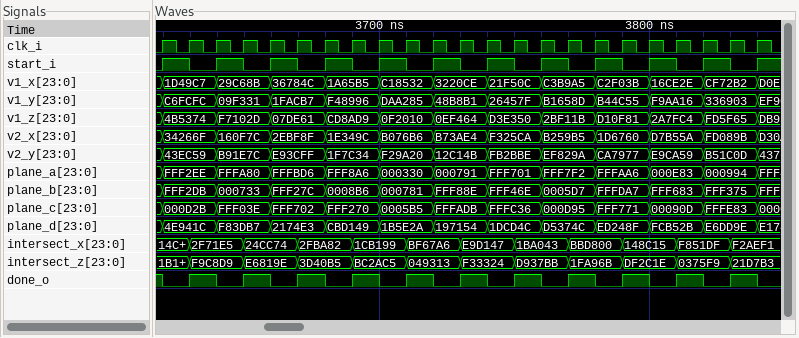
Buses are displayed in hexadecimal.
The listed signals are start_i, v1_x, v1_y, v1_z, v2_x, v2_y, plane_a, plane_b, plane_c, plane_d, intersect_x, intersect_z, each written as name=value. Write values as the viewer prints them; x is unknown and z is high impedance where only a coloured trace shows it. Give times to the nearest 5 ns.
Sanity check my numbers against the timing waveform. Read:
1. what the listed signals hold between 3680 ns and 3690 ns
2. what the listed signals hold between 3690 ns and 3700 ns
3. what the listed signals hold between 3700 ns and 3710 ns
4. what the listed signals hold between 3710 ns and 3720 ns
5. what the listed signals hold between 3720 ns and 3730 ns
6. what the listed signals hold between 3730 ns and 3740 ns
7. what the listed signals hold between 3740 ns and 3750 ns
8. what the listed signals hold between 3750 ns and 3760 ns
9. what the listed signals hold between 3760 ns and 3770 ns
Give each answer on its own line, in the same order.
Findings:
start_i=1, v1_x=1A65B5, v1_y=F48996, v1_z=CD8AD9, v2_x=1E349C, v2_y=1F7C34, plane_a=FFF8A6, plane_b=0008B6, plane_c=FFF270, plane_d=CBD149, intersect_x=2FBA82, intersect_z=3D40B5
start_i=0, v1_x=1A65B5, v1_y=F48996, v1_z=CD8AD9, v2_x=1E349C, v2_y=1F7C34, plane_a=FFF8A6, plane_b=0008B6, plane_c=FFF270, plane_d=CBD149, intersect_x=1CB199, intersect_z=BC2AC5
start_i=1, v1_x=C18532, v1_y=DAA285, v1_z=0F2010, v2_x=B076B6, v2_y=F29A20, plane_a=000330, plane_b=000781, plane_c=0005B5, plane_d=1B5E2A, intersect_x=1CB199, intersect_z=BC2AC5
start_i=0, v1_x=C18532, v1_y=DAA285, v1_z=0F2010, v2_x=B076B6, v2_y=F29A20, plane_a=000330, plane_b=000781, plane_c=0005B5, plane_d=1B5E2A, intersect_x=BF67A6, intersect_z=049313
start_i=1, v1_x=3220CE, v1_y=48B8B1, v1_z=0EF464, v2_x=B73AE4, v2_y=12C14B, plane_a=000791, plane_b=FFF88E, plane_c=FFFADB, plane_d=197154, intersect_x=BF67A6, intersect_z=049313
start_i=0, v1_x=3220CE, v1_y=48B8B1, v1_z=0EF464, v2_x=B73AE4, v2_y=12C14B, plane_a=000791, plane_b=FFF88E, plane_c=FFFADB, plane_d=197154, intersect_x=E9D147, intersect_z=F33324
start_i=1, v1_x=21F50C, v1_y=26457F, v1_z=D3E350, v2_x=F325CA, v2_y=FB2BBE, plane_a=FFF701, plane_b=FFF46E, plane_c=FFFC36, plane_d=1DCD4C, intersect_x=E9D147, intersect_z=F33324
start_i=0, v1_x=21F50C, v1_y=26457F, v1_z=D3E350, v2_x=F325CA, v2_y=FB2BBE, plane_a=FFF701, plane_b=FFF46E, plane_c=FFFC36, plane_d=1DCD4C, intersect_x=1BA043, intersect_z=D937BB
start_i=1, v1_x=C3B9A5, v1_y=B1658D, v1_z=2BF11B, v2_x=B259B5, v2_y=EF829A, plane_a=FFF7F2, plane_b=0005D7, plane_c=000D95, plane_d=D5374C, intersect_x=1BA043, intersect_z=D937BB
